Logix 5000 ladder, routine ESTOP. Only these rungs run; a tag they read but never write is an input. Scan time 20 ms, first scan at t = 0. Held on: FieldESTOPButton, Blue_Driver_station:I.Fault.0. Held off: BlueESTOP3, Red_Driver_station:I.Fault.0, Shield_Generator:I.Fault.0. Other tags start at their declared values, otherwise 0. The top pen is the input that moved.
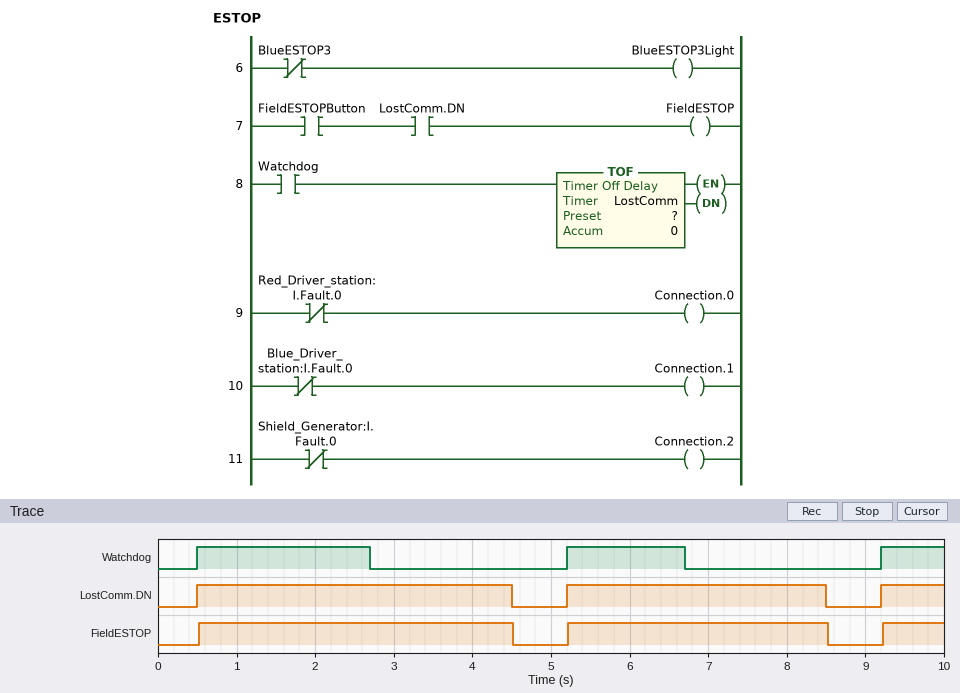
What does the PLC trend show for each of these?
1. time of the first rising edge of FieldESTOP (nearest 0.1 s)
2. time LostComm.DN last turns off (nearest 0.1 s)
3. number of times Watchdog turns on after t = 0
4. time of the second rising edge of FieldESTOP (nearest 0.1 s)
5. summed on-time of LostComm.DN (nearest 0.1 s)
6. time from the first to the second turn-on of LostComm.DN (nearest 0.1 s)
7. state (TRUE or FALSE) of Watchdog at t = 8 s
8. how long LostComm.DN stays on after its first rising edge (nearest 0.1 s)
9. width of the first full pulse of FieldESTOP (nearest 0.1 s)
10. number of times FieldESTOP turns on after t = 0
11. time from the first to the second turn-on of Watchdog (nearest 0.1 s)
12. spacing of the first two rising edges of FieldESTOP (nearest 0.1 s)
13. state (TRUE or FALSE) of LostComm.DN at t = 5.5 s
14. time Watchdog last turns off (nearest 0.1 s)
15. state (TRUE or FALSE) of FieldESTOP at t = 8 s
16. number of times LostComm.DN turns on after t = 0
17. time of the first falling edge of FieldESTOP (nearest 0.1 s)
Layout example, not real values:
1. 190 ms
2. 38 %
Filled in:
1. 0.5 s
2. 8.5 s
3. 3
4. 5.2 s
5. 8.1 s
6. 4.7 s
7. FALSE
8. 4.0 s
9. 4.0 s
10. 3
11. 4.7 s
12. 4.7 s
13. TRUE
14. 6.7 s
15. TRUE
16. 3
17. 4.5 s
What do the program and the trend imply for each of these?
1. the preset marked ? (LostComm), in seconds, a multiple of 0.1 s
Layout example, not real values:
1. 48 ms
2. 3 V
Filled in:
1. 1.8 s
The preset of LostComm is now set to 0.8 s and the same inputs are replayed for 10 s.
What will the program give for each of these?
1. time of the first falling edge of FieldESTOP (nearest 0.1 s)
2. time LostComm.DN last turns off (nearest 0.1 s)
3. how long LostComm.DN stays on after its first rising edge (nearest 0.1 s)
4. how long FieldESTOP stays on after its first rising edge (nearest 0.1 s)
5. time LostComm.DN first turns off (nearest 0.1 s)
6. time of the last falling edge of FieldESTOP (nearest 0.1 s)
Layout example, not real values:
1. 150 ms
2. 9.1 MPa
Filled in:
1. 3.5 s
2. 7.5 s
3. 3.0 s
4. 3.0 s
5. 3.5 s
6. 7.5 s
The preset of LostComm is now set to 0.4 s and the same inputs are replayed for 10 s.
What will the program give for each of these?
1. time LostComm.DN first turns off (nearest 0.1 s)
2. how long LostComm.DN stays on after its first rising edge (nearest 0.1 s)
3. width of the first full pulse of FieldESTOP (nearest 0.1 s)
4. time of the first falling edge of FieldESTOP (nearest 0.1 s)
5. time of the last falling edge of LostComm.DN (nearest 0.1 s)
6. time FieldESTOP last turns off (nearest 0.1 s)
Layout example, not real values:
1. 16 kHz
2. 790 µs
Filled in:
1. 3.1 s
2. 2.6 s
3. 2.6 s
4. 3.1 s
5. 7.1 s
6. 7.1 s
